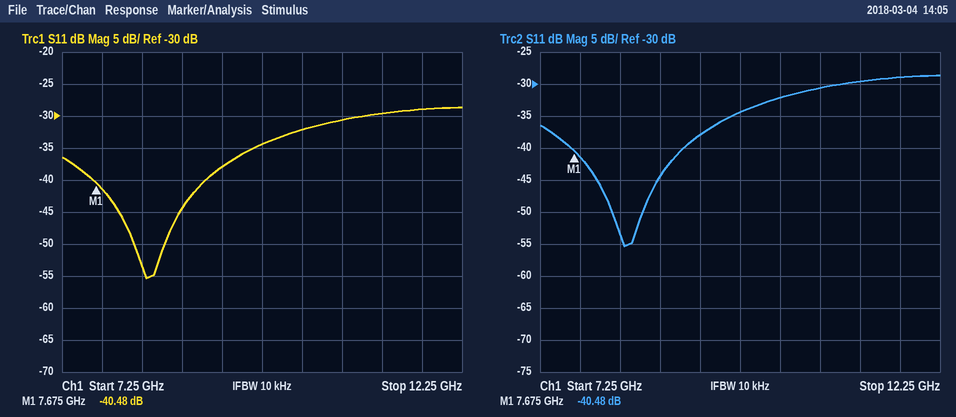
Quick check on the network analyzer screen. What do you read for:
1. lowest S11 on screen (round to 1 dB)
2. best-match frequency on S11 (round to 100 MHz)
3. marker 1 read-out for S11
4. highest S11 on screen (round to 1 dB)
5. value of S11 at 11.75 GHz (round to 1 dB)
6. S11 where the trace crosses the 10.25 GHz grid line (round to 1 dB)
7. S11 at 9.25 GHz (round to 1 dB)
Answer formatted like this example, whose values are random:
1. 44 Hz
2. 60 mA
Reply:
1. -55 dB
2. 8.3 GHz
3. -40.48 dB
4. -29 dB
5. -29 dB
6. -32 dB
7. -38 dB
